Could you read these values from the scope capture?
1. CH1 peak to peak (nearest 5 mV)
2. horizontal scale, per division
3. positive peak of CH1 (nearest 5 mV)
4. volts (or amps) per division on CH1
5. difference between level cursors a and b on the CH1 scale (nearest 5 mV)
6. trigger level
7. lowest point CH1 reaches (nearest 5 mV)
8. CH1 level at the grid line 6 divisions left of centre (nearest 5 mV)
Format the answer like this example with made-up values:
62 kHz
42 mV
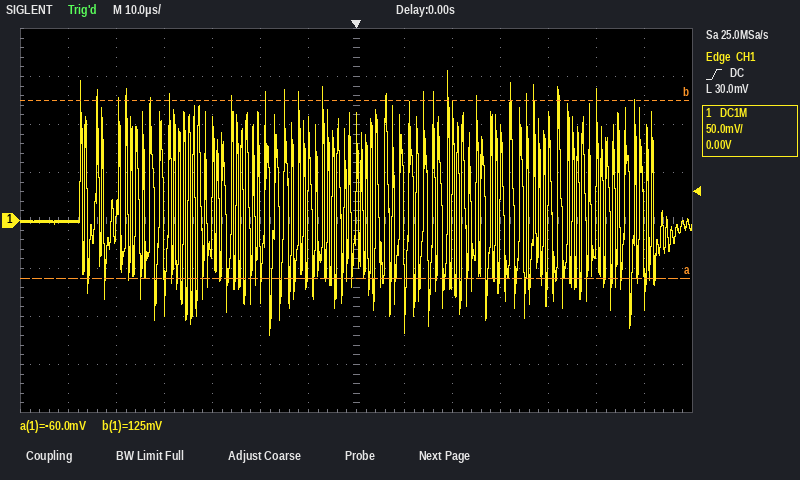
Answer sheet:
275 mV
10 µs
155 mV
50 mV
185 mV
30.0 mV
-120 mV
0 mV
